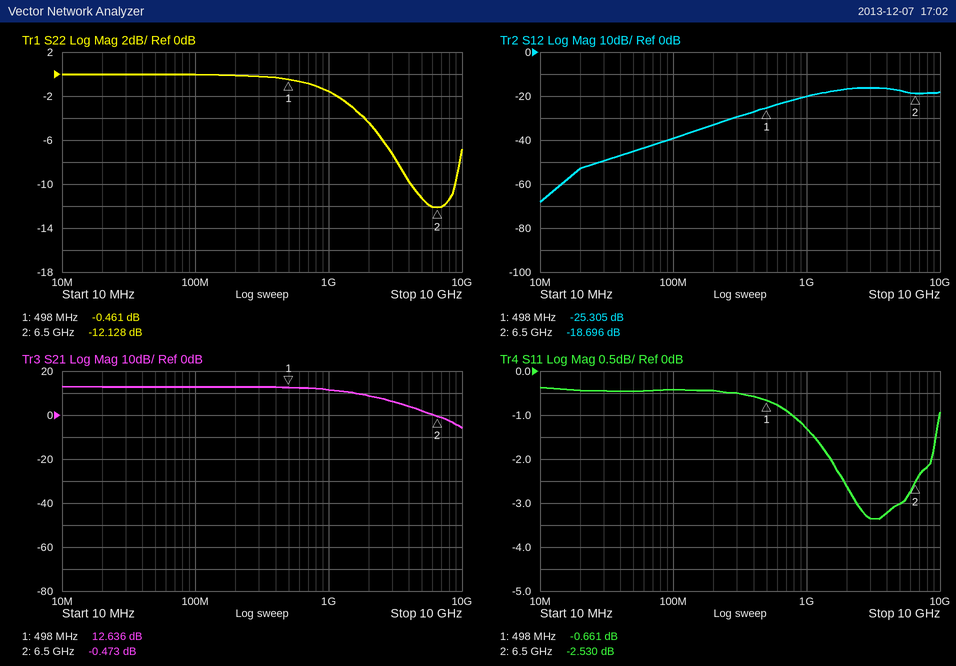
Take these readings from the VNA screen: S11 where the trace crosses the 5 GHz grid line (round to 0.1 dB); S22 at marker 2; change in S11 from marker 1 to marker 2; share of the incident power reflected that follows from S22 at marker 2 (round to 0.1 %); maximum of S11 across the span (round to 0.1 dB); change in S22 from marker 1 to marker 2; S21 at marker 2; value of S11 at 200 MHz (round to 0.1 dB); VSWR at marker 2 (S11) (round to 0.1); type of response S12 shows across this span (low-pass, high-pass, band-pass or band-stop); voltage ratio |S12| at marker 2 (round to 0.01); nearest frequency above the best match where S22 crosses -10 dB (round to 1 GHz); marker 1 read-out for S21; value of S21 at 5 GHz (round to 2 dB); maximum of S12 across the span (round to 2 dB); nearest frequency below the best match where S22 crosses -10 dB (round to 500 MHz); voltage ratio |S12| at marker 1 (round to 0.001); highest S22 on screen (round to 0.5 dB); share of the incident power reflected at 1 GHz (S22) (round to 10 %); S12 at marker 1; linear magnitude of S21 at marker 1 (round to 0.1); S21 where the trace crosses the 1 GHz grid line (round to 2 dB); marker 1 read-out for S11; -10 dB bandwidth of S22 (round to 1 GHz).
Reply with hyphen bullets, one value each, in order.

- -3.0 dB
- -12.128 dB
- -1.869 dB
- 6.1 %
- -0.4 dB
- -11.667 dB
- -0.473 dB
- -0.4 dB
- 6.9
- high-pass
- 0.12
- 9 GHz
- 12.636 dB
- 2 dB
- -16 dB
- 4.0 GHz
- 0.054
- 0.0 dB
- 70 %
- -25.305 dB
- 4.3
- 12 dB
- -0.661 dB
- 5 GHz
